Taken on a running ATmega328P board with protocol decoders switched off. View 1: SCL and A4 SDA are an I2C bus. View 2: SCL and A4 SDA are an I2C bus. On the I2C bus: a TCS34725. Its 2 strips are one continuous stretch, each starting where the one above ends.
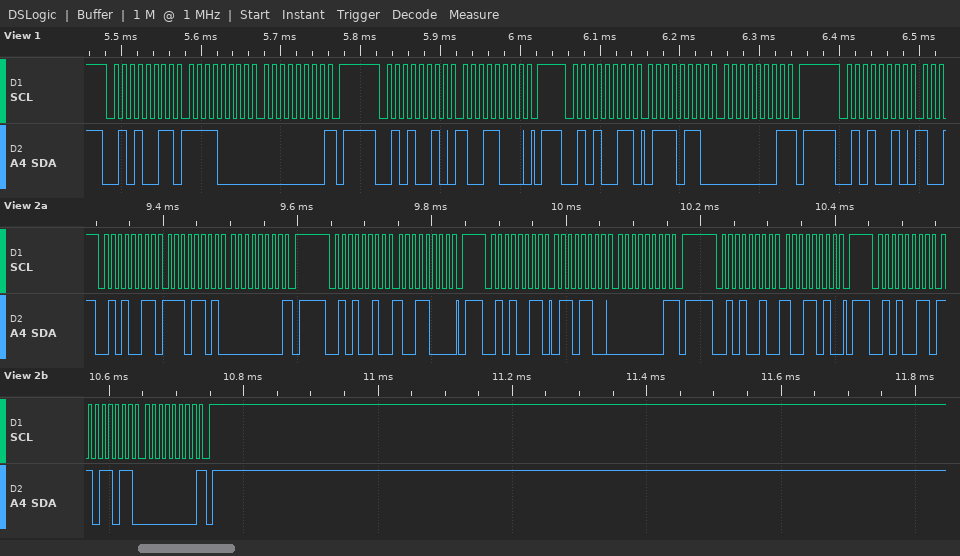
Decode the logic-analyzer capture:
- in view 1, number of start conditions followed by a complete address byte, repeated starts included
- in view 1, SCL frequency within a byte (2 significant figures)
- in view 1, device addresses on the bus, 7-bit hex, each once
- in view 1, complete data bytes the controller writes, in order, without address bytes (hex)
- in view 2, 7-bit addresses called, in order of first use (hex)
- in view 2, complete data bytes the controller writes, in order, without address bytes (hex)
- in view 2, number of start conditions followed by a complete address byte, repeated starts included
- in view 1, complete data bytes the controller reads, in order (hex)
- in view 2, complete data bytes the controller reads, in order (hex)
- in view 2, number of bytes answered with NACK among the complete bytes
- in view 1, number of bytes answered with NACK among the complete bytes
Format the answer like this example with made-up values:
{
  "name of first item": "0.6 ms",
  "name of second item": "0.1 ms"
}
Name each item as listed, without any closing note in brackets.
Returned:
{
  "in view 1, number of start conditions followed by a complete address byte, repeated starts included": "4",
  "in view 1, SCL frequency within a byte": "100 kHz",
  "in view 1, device addresses on the bus, 7-bit hex, each once": "0x29",
  "in view 1, complete data bytes the controller writes, in order, without address bytes": "98",
  "in view 2, 7-bit addresses called, in order of first use": "0x29",
  "in view 2, complete data bytes the controller writes, in order, without address bytes": "98 9A",
  "in view 2, number of start conditions followed by a complete address byte, repeated starts included": "5",
  "in view 1, complete data bytes the controller reads, in order": "F0 00 76 01",
  "in view 2, complete data bytes the controller reads, in order": "ED 00 6C 01 DB 00",
  "in view 2, number of bytes answered with NACK among the complete bytes": "3",
  "in view 1, number of bytes answered with NACK among the complete bytes": "2"
}
